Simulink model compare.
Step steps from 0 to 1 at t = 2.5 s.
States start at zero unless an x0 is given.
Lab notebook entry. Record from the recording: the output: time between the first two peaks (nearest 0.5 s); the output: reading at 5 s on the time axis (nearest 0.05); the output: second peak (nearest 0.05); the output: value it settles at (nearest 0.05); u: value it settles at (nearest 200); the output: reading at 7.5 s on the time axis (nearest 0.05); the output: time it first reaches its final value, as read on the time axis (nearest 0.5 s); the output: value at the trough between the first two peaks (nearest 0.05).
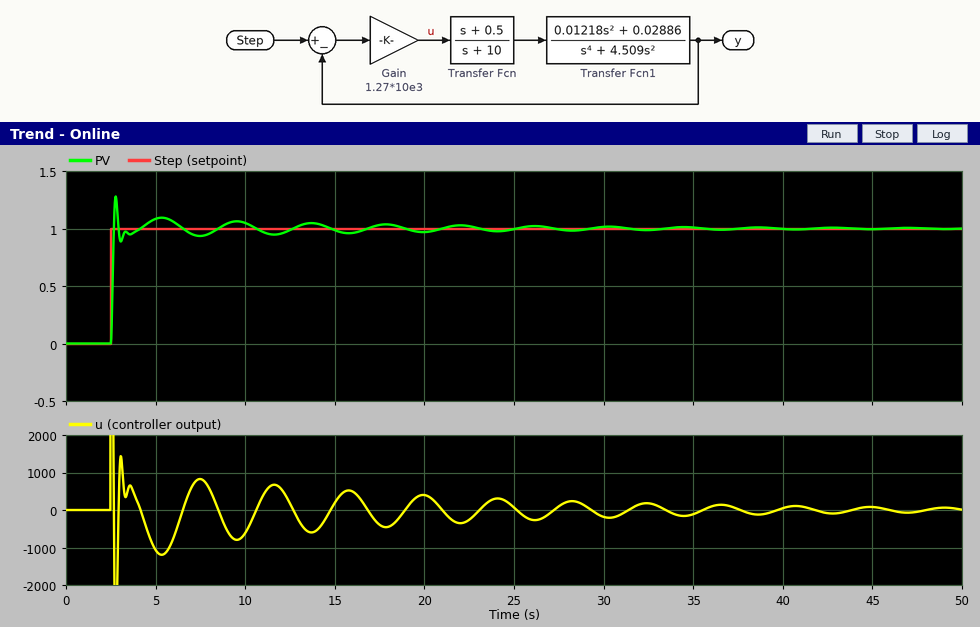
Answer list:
2.5 s
1.10
1.10
1.00
0
0.95
2.5 s
0.90
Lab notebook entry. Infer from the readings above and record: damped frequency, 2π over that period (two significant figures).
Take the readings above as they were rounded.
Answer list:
2.5 rad/s
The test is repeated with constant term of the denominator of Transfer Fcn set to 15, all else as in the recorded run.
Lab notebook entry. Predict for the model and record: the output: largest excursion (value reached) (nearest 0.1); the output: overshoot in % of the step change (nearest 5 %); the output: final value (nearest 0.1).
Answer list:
1.1
15 %
1.0
